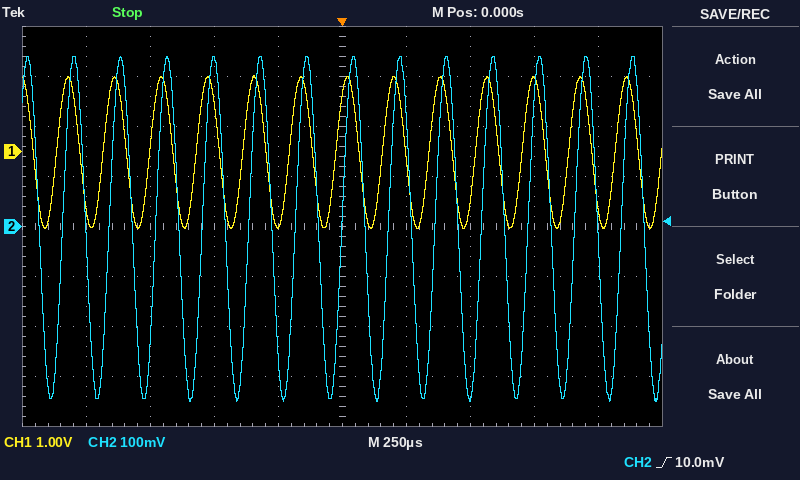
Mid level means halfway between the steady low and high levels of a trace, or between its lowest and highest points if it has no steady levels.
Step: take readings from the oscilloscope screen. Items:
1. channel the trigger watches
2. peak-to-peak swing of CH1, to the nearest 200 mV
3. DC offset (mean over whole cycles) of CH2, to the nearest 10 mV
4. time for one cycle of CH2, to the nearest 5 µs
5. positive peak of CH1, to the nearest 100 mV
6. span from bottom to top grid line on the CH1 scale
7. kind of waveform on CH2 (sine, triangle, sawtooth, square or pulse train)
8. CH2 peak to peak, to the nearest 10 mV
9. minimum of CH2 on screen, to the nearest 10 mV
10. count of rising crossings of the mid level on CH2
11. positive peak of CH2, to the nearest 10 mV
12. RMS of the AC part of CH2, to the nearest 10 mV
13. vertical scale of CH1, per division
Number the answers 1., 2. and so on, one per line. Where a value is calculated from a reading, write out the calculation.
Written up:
1. CH2
2. 3.0 V
3. (340 mV + (-350 mV)) / 2 ≈ 0 mV
4. 180 µs
5. 1.5 V
6. 8 V
7. sine
8. 340 mV − (-350 mV) = 690 mV
9. -350 mV
10. 13
11. 340 mV
12. 690 mV / (2√2) ≈ 244 mV, so 240 mV to the nearest 10 mV
13. 1 V
